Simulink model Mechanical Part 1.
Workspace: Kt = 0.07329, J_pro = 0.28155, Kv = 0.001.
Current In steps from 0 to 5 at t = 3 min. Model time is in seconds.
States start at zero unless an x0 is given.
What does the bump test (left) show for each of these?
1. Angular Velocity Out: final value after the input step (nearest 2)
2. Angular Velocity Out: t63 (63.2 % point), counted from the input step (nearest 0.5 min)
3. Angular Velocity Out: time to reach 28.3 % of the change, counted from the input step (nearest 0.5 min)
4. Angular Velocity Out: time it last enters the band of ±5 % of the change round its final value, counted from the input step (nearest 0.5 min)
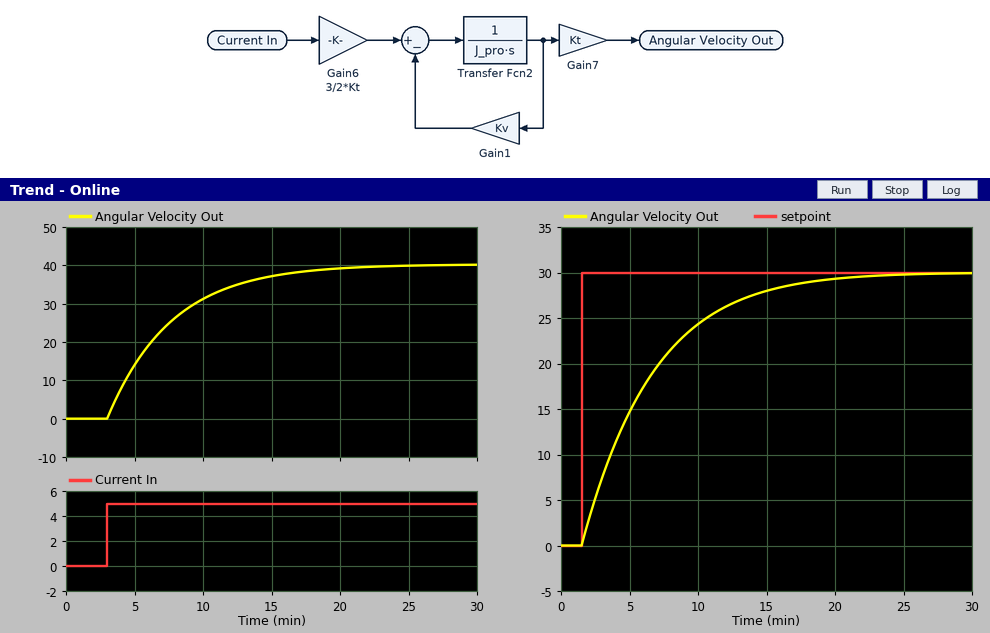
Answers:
40
4.5 min
1.5 min
14.0 min
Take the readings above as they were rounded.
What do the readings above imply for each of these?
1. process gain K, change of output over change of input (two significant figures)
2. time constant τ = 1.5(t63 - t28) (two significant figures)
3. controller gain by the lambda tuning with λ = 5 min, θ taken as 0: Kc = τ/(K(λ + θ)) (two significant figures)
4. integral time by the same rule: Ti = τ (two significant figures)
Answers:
8.0
4.5 min
0.11
4.5 min
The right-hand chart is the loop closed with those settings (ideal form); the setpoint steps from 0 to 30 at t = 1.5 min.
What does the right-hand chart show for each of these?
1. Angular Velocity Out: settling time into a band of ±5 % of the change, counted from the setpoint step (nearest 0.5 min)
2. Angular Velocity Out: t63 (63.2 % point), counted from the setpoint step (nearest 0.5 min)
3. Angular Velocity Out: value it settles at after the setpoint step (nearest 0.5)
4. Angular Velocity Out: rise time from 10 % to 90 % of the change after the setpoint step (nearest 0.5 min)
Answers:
15.0 min
5.0 min
30.0
11.0 min
